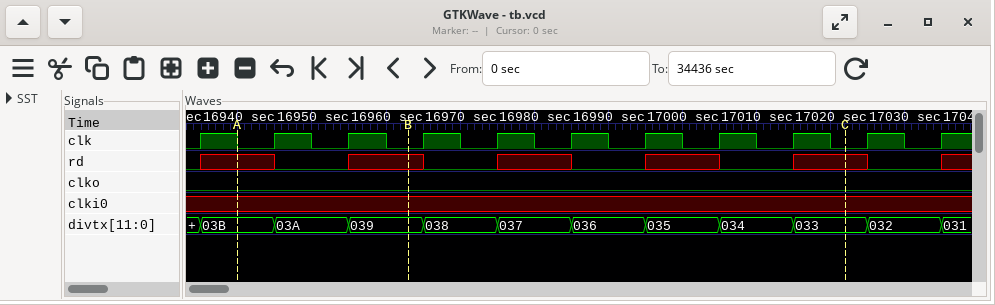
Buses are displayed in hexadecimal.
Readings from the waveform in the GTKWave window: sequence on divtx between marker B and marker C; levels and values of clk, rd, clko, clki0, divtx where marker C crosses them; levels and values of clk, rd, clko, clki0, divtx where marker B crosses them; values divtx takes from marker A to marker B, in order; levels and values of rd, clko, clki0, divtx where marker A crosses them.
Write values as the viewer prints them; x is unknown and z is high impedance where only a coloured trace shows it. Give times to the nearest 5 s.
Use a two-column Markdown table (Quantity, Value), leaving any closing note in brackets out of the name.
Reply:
| Quantity | Value |
|---|---|
| sequence on divtx between marker B and marker C | 039, 038, 037, 036, 035, 034, 033 |
| levels and values of clk, rd, clko, clki0, divtx where marker C crosses them | clk=0, rd=x, clko=0, clki0=x, divtx=033 |
| levels and values of clk, rd, clko, clki0, divtx where marker B crosses them | clk=0, rd=x, clko=0, clki0=x, divtx=039 |
| values divtx takes from marker A to marker B, in order | 03B, 03A, 039 |
| levels and values of rd, clko, clki0, divtx where marker A crosses them | rd=x, clko=0, clki0=x, divtx=03B |
